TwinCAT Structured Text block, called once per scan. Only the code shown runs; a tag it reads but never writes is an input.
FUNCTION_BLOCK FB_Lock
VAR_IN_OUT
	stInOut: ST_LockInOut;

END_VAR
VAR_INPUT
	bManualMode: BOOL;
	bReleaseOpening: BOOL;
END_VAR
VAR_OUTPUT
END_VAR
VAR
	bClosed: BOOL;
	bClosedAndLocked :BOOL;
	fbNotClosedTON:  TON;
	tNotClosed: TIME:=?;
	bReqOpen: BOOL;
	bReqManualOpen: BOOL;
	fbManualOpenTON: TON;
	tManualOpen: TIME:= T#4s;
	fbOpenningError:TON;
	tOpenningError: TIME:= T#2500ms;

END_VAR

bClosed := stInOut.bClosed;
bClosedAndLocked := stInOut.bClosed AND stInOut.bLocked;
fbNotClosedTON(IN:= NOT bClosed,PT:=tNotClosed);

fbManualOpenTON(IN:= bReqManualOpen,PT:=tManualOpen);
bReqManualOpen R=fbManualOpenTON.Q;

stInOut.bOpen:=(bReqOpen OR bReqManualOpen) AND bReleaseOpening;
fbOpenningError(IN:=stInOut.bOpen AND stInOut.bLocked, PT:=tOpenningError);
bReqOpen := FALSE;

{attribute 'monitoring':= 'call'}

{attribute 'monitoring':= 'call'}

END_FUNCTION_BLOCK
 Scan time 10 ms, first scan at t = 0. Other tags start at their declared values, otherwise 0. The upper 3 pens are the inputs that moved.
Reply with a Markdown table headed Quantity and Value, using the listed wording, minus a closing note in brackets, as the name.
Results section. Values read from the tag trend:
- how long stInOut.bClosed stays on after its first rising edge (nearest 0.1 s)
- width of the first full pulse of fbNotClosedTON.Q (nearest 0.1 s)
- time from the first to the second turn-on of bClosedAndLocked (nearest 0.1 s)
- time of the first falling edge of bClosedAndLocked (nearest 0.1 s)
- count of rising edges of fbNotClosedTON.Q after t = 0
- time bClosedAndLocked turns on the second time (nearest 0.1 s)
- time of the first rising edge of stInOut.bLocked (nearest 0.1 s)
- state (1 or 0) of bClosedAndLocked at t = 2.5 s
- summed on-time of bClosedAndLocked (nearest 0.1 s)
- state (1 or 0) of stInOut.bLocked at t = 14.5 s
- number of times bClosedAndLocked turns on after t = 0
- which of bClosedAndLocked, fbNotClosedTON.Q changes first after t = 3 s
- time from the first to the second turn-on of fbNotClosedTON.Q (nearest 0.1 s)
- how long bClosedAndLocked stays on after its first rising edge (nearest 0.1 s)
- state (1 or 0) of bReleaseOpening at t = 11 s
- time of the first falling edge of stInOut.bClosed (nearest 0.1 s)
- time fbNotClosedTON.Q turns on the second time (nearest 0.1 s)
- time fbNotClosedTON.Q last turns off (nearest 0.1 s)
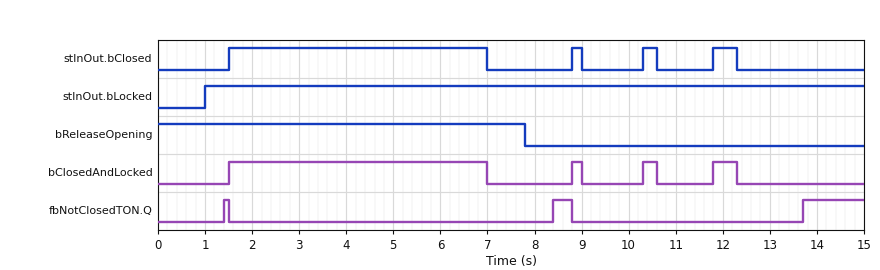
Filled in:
| Quantity | Value |
|---|---|
| how long stInOut.bClosed stays on after its first rising edge | 5.5 s |
| width of the first full pulse of fbNotClosedTON.Q | 0.1 s |
| time from the first to the second turn-on of bClosedAndLocked | 7.3 s |
| time of the first falling edge of bClosedAndLocked | 7.0 s |
| count of rising edges of fbNotClosedTON.Q after t = 0 | 3 |
| time bClosedAndLocked turns on the second time | 8.8 s |
| time of the first rising edge of stInOut.bLocked | 1.0 s |
| state (1 or 0) of bClosedAndLocked at t = 2.5 s | 1 |
| summed on-time of bClosedAndLocked | 6.5 s |
| state (1 or 0) of stInOut.bLocked at t = 14.5 s | 1 |
| number of times bClosedAndLocked turns on after t = 0 | 4 |
| which of bClosedAndLocked, fbNotClosedTON.Q changes first after t = 3 s | bClosedAndLocked |
| time from the first to the second turn-on of fbNotClosedTON.Q | 7.0 s |
| how long bClosedAndLocked stays on after its first rising edge | 5.5 s |
| state (1 or 0) of bReleaseOpening at t = 11 s | 0 |
| time of the first falling edge of stInOut.bClosed | 7.0 s |
| time fbNotClosedTON.Q turns on the second time | 8.4 s |
| time fbNotClosedTON.Q last turns off | 8.8 s |
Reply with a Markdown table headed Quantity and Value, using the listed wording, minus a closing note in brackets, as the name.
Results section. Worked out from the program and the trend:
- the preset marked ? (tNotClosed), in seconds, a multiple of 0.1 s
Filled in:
| Quantity | Value |
|---|---|
| the preset marked ? (tNotClosed), in seconds, a multiple of 0.1 s | 1.4 s |
